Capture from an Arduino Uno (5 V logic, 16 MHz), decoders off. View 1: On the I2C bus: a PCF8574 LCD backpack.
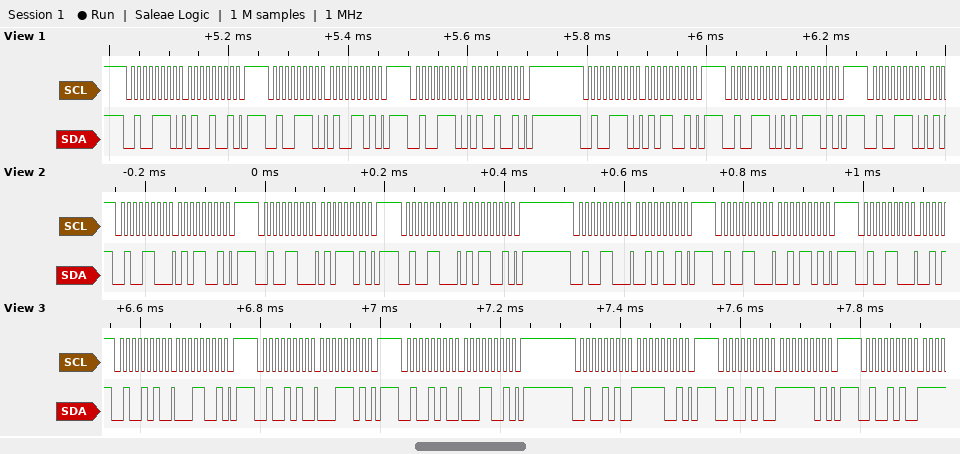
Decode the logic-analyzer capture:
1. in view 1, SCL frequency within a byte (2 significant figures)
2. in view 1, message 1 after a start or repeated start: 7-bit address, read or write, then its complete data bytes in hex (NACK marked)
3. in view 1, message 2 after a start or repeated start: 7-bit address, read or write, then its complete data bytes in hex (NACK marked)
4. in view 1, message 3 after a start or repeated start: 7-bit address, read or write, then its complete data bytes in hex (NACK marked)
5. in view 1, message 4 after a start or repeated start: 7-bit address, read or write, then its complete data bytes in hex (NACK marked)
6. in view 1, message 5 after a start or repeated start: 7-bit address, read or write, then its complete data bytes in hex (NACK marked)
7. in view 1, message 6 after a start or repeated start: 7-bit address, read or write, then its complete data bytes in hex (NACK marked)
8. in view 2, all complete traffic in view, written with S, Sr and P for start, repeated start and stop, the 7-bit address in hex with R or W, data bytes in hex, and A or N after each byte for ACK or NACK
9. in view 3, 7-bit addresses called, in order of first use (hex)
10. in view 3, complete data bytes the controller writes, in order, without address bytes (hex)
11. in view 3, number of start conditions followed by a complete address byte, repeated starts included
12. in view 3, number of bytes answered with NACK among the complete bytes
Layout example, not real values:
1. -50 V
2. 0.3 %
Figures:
1. 100 kHz
2. 0x27 write: 49
3. 0x27 write: 4D
4. 0x27 write: 49
5. 0x27 write: 59
6. 0x27 write: 5D
7. 0x27 write
8. S 26W A 59 A P S 26W A 5D A P S 26W A 59 A P S 26W A 29 A P S 26W A 2D A P S 26W A
9. 0x25
10. 19 1D 19 F9 FD
11. 6
12. 0
